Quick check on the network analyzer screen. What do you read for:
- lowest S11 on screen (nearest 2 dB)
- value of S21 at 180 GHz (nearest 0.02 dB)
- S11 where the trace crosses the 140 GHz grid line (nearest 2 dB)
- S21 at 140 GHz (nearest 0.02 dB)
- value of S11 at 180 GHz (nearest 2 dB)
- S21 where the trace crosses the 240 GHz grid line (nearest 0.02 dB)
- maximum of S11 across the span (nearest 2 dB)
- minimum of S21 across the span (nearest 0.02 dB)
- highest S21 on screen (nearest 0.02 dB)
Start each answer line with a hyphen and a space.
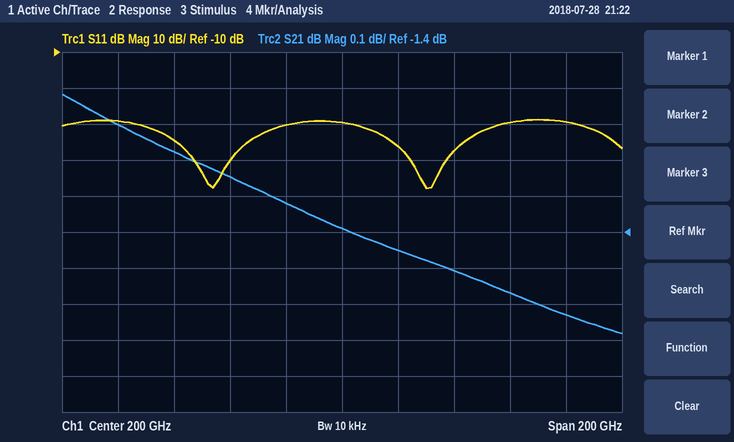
- -48 dB
- -1.32 dB
- -34 dB
- -1.18 dB
- -30 dB
- -1.50 dB
- -28 dB
- -1.68 dB
- -1.02 dB
